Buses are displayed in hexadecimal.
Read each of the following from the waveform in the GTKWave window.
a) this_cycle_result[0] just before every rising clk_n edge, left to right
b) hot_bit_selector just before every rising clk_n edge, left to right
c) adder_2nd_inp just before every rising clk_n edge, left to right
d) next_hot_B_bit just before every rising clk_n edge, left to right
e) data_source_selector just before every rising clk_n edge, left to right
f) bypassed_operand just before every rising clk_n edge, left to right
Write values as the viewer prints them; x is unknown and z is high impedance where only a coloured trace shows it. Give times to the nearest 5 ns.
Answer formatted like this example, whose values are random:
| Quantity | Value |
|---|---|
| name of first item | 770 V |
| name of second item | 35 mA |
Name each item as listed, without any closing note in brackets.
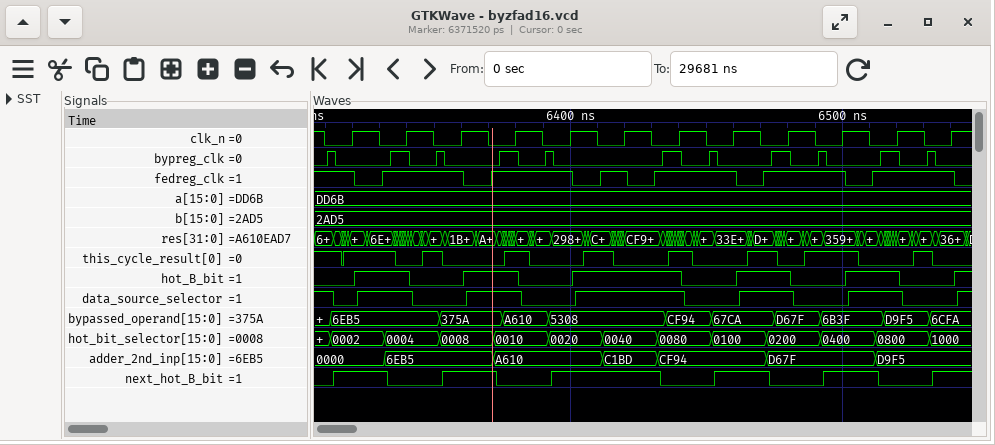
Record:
| Quantity | Value |
|---|---|
| this_cycle_result[0] just before every rising clk_n edge, left to right | 1 0 0 1 0 0 1 0 0 1 0 0 |
| hot_bit_selector just before every rising clk_n edge, left to right | 0002, 0004, 0008, 0010, 0020, 0040, 0080, 0100, 0200, 0400, 0800, 1000 |
| adder_2nd_inp just before every rising clk_n edge, left to right | 0000, 6EB5, 6EB5, A610, A610, C1BD, CF94, CF94, D67F, D67F, D9F5, D9F5 |
| next_hot_B_bit just before every rising clk_n edge, left to right | 1 0 1 0 1 1 0 1 0 1 0 1 |
| data_source_selector just before every rising clk_n edge, left to right | 0 1 0 1 0 1 1 0 1 0 1 0 |
| bypassed_operand just before every rising clk_n edge, left to right | 6EB5, 6EB5, 375A, A610, 5308, 5308, CF94, 67CA, D67F, 6B3F, D9F5, 6CFA |
